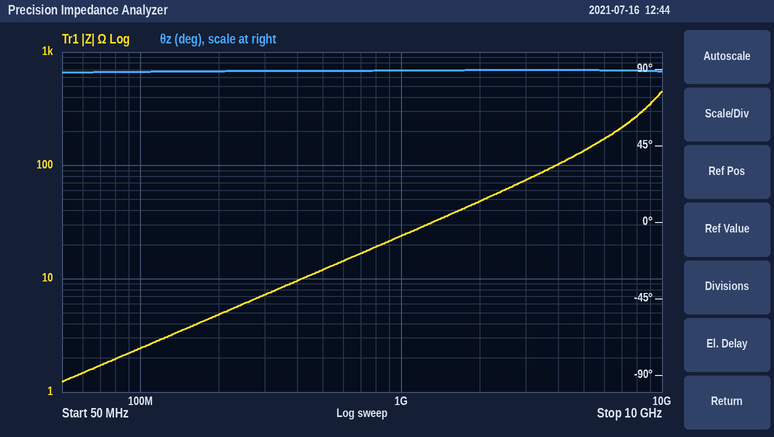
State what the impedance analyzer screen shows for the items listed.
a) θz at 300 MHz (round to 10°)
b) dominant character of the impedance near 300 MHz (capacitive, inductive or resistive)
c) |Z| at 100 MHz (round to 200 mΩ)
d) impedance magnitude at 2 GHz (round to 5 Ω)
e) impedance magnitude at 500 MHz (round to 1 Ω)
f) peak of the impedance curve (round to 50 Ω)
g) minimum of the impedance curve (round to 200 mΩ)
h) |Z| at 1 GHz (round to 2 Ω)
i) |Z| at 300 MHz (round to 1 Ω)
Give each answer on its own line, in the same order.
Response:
90°
inductive
2.4 Ω
50 Ω
12 Ω
450 Ω
1.2 Ω
24 Ω
7 Ω
